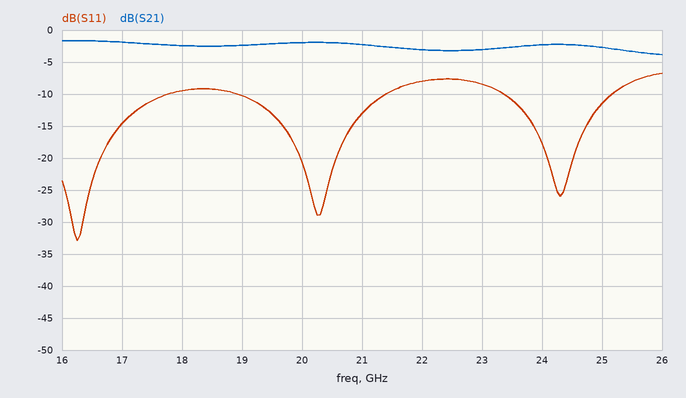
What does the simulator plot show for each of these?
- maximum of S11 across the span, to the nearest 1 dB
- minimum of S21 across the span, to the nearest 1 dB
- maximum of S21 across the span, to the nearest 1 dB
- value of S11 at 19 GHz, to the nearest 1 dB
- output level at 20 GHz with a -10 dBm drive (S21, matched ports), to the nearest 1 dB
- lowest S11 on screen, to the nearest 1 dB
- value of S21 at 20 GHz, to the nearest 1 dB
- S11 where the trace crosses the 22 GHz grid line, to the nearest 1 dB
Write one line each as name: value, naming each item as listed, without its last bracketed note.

maximum of S11 across the span, to the nearest 1 dB: -7 dB
minimum of S21 across the span, to the nearest 1 dB: -4 dB
maximum of S21 across the span, to the nearest 1 dB: -2 dB
value of S11 at 19 GHz, to the nearest 1 dB: -10 dB
output level at 20 GHz with a -10 dBm drive (S21, matched ports), to the nearest 1 dB: -12 dBm
lowest S11 on screen, to the nearest 1 dB: -33 dB
value of S21 at 20 GHz, to the nearest 1 dB: -2 dB
S11 where the trace crosses the 22 GHz grid line, to the nearest 1 dB: -8 dB
